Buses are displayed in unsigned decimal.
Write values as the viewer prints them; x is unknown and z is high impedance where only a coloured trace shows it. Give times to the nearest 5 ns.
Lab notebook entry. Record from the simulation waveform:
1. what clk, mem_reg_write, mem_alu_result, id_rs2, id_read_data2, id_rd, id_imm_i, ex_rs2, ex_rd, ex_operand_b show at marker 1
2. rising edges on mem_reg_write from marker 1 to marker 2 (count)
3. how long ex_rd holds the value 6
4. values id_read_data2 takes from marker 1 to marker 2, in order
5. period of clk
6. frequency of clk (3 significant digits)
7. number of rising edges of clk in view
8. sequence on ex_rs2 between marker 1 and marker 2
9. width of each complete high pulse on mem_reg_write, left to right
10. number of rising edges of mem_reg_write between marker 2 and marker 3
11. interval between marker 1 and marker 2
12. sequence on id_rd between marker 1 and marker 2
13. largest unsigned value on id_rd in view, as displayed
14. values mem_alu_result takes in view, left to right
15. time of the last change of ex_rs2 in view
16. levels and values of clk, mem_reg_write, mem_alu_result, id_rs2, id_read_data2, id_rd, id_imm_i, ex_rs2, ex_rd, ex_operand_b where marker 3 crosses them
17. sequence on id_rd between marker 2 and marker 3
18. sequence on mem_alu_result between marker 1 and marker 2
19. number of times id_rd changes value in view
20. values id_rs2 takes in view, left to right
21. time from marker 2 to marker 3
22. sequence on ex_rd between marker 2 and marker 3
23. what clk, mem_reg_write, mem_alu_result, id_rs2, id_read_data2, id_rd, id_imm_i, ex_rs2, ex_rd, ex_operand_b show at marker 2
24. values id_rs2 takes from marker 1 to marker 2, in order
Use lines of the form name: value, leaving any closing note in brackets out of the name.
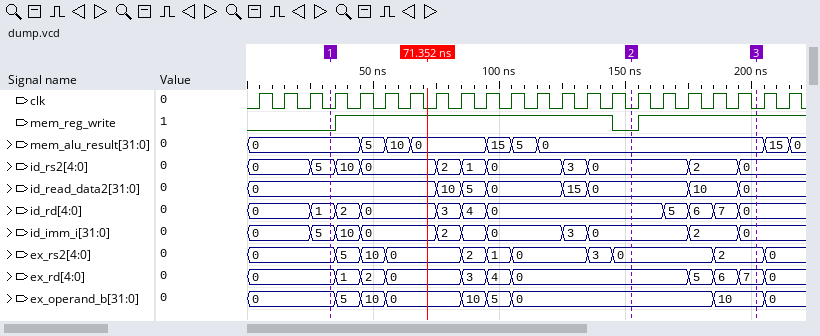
what clk, mem_reg_write, mem_alu_result, id_rs2, id_read_data2, id_rd, id_imm_i, ex_rs2, ex_rd, ex_operand_b show at marker 1: clk=0, mem_reg_write=0, mem_alu_result=0, id_rs2=5, id_read_data2=0, id_rd=1, id_imm_i=5, ex_rs2=0, ex_rd=0, ex_operand_b=0
rising edges on mem_reg_write from marker 1 to marker 2: 1
how long ex_rd holds the value 6: 10 ns
values id_read_data2 takes from marker 1 to marker 2, in order: 0, 10, 5, 0, 15, 0
period of clk: 10 ns
frequency of clk: 100 MHz
number of rising edges of clk in view: 22
sequence on ex_rs2 between marker 1 and marker 2: 0, 5, 10, 0, 2, 1, 0, 3, 0
width of each complete high pulse on mem_reg_write, left to right: 110 ns
number of rising edges of mem_reg_write between marker 2 and marker 3: 1
interval between marker 1 and marker 2: 120 ns
sequence on id_rd between marker 1 and marker 2: 1, 2, 0, 3, 4, 0
largest unsigned value on id_rd in view, as displayed: 7
values mem_alu_result takes in view, left to right: 0, 5, 10, 0, 15, 5, 0, 15, 0
time of the last change of ex_rs2 in view: 205 ns
levels and values of clk, mem_reg_write, mem_alu_result, id_rs2, id_read_data2, id_rd, id_imm_i, ex_rs2, ex_rd, ex_operand_b where marker 3 crosses them: clk=0, mem_reg_write=1, mem_alu_result=0, id_rs2=0, id_read_data2=0, id_rd=0, id_imm_i=0, ex_rs2=2, ex_rd=7, ex_operand_b=10
sequence on id_rd between marker 2 and marker 3: 0, 5, 6, 7, 0
sequence on mem_alu_result between marker 1 and marker 2: 0, 5, 10, 0, 15, 5, 0
number of times id_rd changes value in view: 10
values id_rs2 takes in view, left to right: 0, 5, 10, 0, 2, 1, 0, 3, 0, 2, 0
time from marker 2 to marker 3: 50 ns
sequence on ex_rd between marker 2 and marker 3: 0, 5, 6, 7
what clk, mem_reg_write, mem_alu_result, id_rs2, id_read_data2, id_rd, id_imm_i, ex_rs2, ex_rd, ex_operand_b show at marker 2: clk=0, mem_reg_write=0, mem_alu_result=0, id_rs2=0, id_read_data2=0, id_rd=0, id_imm_i=0, ex_rs2=0, ex_rd=0, ex_operand_b=0
values id_rs2 takes from marker 1 to marker 2, in order: 5, 10, 0, 2, 1, 0, 3, 0
